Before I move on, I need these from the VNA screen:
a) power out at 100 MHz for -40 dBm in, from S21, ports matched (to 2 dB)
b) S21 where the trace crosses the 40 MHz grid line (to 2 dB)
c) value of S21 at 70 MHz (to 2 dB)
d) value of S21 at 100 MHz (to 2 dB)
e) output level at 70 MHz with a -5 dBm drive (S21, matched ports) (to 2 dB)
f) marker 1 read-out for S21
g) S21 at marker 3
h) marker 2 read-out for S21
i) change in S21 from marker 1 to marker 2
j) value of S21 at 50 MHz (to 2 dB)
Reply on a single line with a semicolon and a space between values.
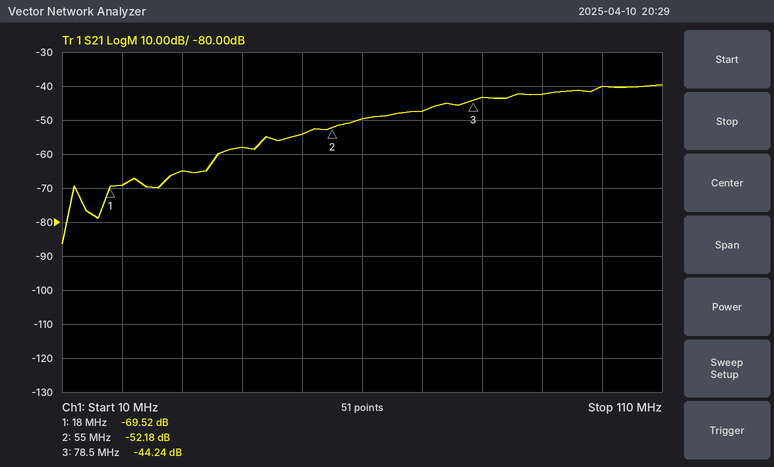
-80 dBm; -58 dB; -48 dB; -40 dB; -52 dBm; -69.52 dB; -44.24 dB; -52.18 dB; 17.34 dB; -54 dB
